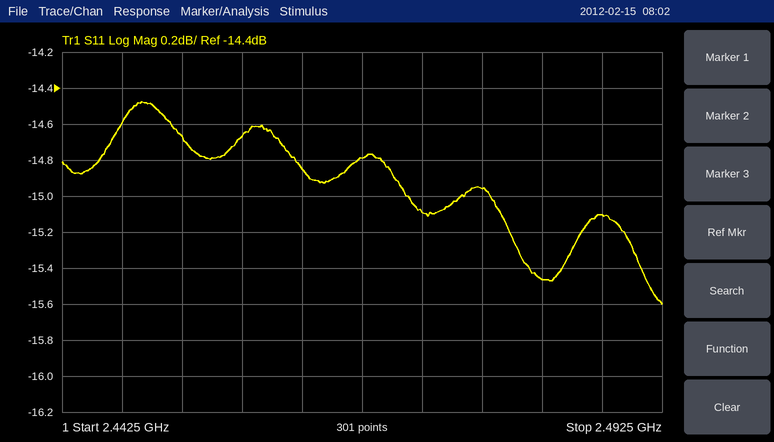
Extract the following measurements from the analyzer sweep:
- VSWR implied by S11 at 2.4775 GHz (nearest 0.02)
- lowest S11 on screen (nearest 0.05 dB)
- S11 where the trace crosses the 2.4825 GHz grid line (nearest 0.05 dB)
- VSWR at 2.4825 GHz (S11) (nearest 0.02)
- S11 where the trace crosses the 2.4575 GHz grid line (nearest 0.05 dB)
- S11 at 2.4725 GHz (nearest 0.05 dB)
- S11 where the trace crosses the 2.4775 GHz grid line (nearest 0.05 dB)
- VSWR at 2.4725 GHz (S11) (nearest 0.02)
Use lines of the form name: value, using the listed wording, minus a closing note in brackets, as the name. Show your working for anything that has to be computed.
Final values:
VSWR implied by S11 at 2.4775 GHz: |Γ| = 10^(-14.95/20) = 0.1789; VSWR = (1 + 0.1789)/(1 − 0.1789) ≈ 1.44
lowest S11 on screen: -15.60 dB
S11 where the trace crosses the 2.4825 GHz grid line: -15.45 dB
VSWR at 2.4825 GHz (S11): |Γ| = 10^(-15.45/20) = 0.1688; VSWR = (1 + 0.1688)/(1 − 0.1688) ≈ 1.41, so 1.40 to the nearest 0.02
S11 where the trace crosses the 2.4575 GHz grid line: -14.65 dB
S11 at 2.4725 GHz: -15.10 dB
S11 where the trace crosses the 2.4775 GHz grid line: -14.95 dB
VSWR at 2.4725 GHz (S11): |Γ| = 10^(-15.1/20) = 0.1758; VSWR = (1 + 0.1758)/(1 − 0.1758) ≈ 1.43, so 1.42 to the nearest 0.02
